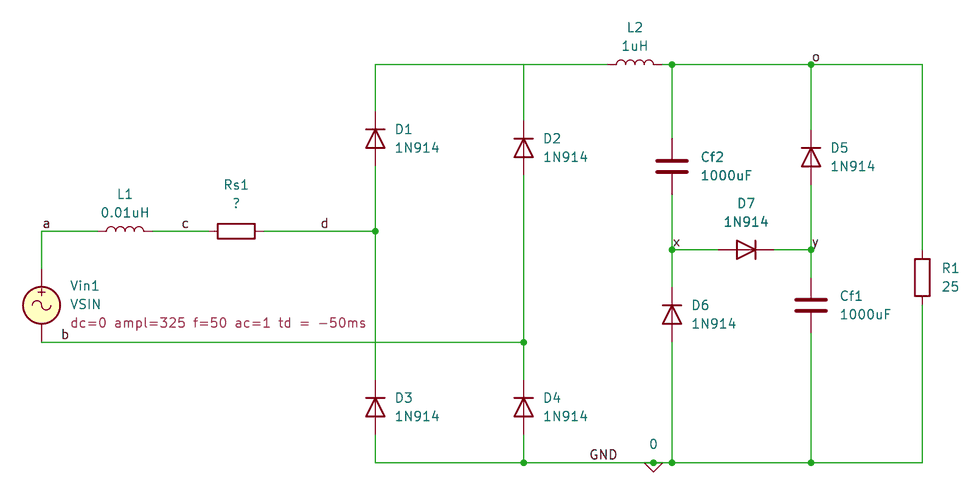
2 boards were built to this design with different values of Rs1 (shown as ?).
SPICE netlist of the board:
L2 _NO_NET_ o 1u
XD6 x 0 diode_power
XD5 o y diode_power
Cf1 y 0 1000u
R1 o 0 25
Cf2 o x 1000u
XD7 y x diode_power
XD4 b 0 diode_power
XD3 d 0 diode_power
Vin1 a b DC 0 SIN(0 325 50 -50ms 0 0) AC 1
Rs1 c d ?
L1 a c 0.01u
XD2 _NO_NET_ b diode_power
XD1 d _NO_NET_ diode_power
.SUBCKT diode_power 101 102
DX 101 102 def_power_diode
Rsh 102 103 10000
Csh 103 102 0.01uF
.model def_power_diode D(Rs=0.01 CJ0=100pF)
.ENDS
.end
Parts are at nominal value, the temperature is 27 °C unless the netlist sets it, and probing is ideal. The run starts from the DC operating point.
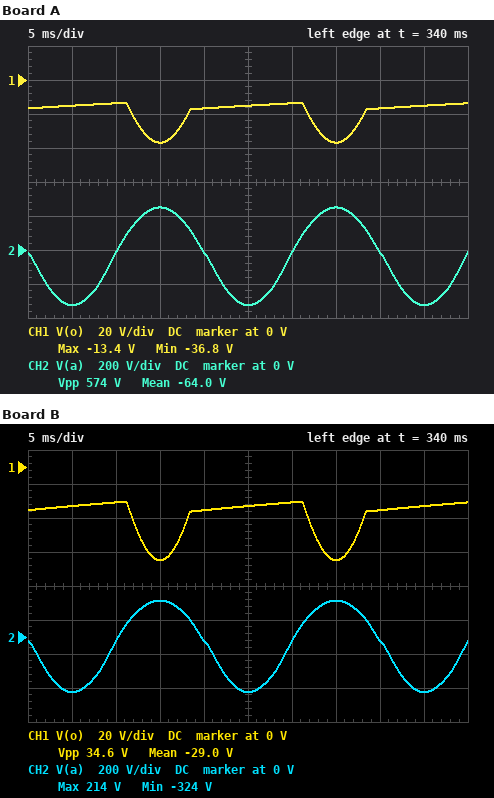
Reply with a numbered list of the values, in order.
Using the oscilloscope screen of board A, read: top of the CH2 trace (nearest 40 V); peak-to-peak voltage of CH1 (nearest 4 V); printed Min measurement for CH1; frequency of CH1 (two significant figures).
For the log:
1. 240 V
2. 24 V
3. -36.8 V
4. 50 Hz
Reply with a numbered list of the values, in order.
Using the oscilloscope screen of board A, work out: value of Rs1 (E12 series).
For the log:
1. 0.068 Ω
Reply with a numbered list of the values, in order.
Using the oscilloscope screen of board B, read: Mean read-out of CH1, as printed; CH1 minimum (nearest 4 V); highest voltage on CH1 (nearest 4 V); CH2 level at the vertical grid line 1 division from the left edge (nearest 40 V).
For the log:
1. -29.0 V
2. -56 V
3. -20 V
4. -320 V
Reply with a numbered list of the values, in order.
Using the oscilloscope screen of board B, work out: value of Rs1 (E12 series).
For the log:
1. 0.039 Ω
